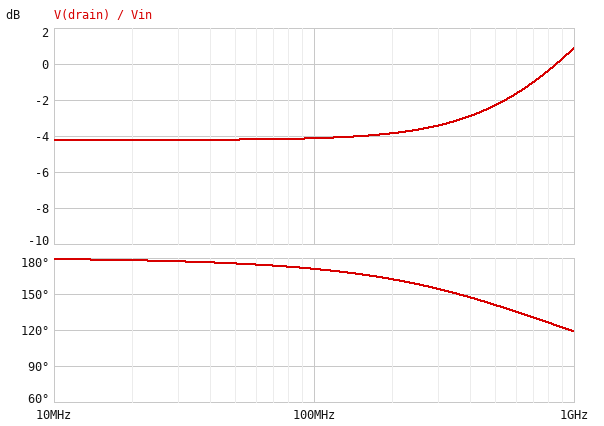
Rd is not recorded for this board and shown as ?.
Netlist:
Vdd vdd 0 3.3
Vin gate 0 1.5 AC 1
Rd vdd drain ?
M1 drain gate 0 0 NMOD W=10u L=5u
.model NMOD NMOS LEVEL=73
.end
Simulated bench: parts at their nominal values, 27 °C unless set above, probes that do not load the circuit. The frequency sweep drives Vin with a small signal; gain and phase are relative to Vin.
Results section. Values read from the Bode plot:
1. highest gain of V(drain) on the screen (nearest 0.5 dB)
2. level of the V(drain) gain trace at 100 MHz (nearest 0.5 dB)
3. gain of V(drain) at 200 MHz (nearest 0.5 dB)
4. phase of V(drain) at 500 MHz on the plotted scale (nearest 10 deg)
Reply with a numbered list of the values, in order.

1. 1.0 dB
2. -4.0 dB
3. -4.0 dB
4. 140 deg
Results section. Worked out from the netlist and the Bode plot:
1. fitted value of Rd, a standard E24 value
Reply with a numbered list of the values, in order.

1. 2.7 kΩ
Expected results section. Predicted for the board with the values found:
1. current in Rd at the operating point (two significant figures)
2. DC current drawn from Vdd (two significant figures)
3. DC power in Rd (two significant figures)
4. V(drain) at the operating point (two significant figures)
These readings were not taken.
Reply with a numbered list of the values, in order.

1. 110 µA
2. 110 µA
3. 32 µW
4. 3.0 V
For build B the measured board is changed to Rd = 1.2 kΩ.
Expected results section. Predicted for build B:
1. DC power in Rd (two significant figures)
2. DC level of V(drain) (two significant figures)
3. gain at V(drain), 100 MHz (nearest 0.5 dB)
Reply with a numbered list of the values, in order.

1. 14 µW
2. 3.2 V
3. -11.0 dB
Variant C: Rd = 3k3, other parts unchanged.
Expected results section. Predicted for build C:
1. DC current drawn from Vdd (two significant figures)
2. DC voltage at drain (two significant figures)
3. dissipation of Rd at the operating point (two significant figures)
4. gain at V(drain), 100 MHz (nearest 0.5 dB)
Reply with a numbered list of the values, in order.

1. 110 µA
2. 2.9 V
3. 39 µW
4. -2.5 dB
